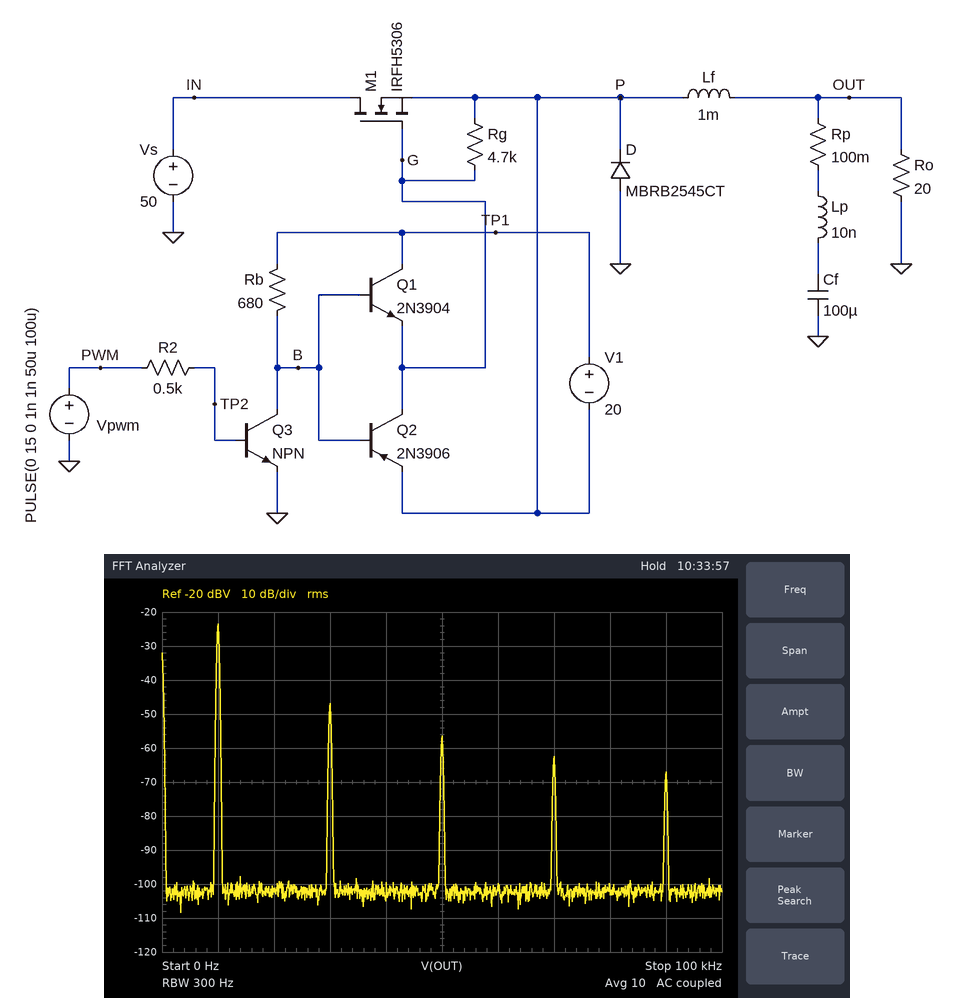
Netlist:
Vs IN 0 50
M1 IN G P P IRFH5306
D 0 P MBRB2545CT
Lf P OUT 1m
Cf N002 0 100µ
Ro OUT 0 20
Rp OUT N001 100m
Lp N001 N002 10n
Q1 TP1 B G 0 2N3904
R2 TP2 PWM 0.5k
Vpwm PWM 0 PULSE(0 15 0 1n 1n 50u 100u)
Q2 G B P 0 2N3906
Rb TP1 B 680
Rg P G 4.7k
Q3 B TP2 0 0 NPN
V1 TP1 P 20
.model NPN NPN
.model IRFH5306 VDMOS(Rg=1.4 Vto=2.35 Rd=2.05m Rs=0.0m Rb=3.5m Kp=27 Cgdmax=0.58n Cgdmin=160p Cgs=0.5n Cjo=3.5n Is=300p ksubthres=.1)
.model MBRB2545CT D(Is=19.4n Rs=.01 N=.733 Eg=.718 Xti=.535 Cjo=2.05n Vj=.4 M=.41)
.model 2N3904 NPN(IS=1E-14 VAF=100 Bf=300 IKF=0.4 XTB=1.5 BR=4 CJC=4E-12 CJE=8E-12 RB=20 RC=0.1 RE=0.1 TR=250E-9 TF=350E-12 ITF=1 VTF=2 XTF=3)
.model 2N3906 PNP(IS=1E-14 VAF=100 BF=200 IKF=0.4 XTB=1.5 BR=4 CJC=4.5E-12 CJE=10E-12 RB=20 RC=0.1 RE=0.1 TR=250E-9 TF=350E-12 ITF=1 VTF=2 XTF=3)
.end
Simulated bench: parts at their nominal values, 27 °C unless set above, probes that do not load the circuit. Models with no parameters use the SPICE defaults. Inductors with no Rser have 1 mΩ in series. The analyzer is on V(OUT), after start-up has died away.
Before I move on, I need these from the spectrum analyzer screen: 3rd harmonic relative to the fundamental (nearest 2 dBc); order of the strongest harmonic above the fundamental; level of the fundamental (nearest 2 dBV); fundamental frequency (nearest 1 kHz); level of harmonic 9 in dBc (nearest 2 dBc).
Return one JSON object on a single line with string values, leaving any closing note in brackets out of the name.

{"3rd harmonic relative to the fundamental": "-24 dBc", "order of the strongest harmonic above the fundamental": "3", "level of the fundamental": "-24 dBV", "fundamental frequency": "10 kHz", "level of harmonic 9 in dBc": "-44 dBc"}
